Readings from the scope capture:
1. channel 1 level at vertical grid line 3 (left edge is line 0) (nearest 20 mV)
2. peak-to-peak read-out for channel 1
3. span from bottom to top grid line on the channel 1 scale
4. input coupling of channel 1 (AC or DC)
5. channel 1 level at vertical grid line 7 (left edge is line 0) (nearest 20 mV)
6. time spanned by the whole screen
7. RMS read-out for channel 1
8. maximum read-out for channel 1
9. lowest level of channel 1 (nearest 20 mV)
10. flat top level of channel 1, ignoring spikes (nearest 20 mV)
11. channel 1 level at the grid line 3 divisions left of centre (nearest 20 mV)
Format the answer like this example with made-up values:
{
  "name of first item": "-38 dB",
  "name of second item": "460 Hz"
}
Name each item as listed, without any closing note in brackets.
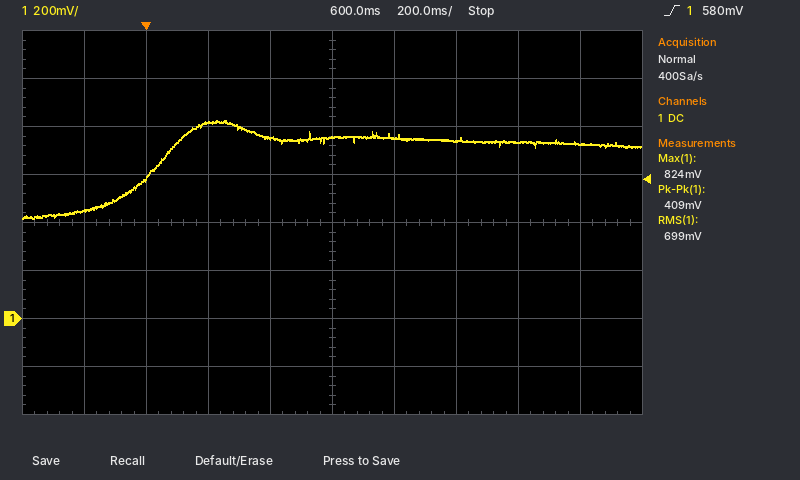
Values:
{
  "channel 1 level at vertical grid line 3 (left edge is line 0)": "820 mV",
  "peak-to-peak read-out for channel 1": "409 mV",
  "span from bottom to top grid line on the channel 1 scale": "1.6 V",
  "input coupling of channel 1": "DC",
  "channel 1 level at vertical grid line 7 (left edge is line 0)": "740 mV",
  "time spanned by the whole screen": "2 s",
  "RMS read-out for channel 1": "699 mV",
  "maximum read-out for channel 1": "824 mV",
  "lowest level of channel 1": "420 mV",
  "flat top level of channel 1, ignoring spikes": "740 mV",
  "channel 1 level at the grid line 3 divisions left of centre": "580 mV"
}
